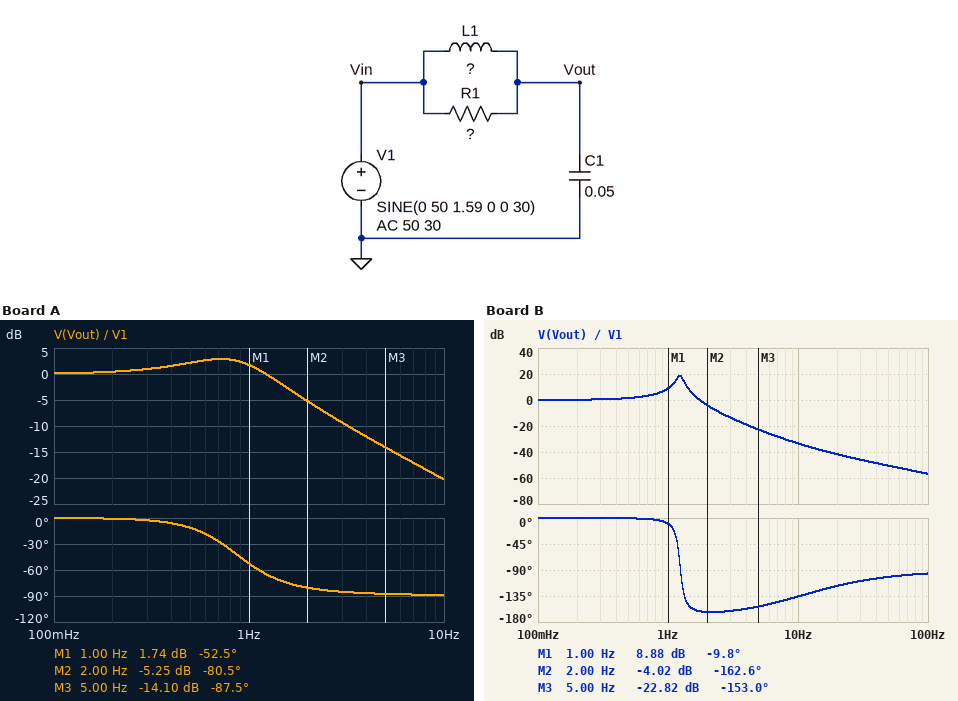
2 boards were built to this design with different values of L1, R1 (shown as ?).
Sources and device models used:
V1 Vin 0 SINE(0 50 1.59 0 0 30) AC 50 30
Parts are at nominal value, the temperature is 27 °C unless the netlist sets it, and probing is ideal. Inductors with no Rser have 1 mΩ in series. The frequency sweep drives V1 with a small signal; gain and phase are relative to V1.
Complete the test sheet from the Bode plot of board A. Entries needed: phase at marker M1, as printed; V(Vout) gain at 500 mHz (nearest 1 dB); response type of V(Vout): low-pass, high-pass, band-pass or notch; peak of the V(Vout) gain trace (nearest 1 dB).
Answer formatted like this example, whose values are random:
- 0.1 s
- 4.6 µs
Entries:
- -52.5 deg
- 2 dB
- low-pass
- 3 dB
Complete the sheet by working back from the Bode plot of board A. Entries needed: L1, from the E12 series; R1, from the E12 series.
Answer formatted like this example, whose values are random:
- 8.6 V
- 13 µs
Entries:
- 680 mH
- 3.3 Ω
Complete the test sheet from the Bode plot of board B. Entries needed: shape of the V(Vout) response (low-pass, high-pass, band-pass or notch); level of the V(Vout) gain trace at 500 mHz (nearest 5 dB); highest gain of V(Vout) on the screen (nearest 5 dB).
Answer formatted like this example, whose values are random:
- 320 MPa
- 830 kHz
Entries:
- low-pass
- 0 dB
- 20 dB
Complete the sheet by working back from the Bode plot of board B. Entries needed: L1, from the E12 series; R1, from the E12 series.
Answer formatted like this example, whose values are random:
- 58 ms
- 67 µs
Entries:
- 330 mH
- 22 Ω
